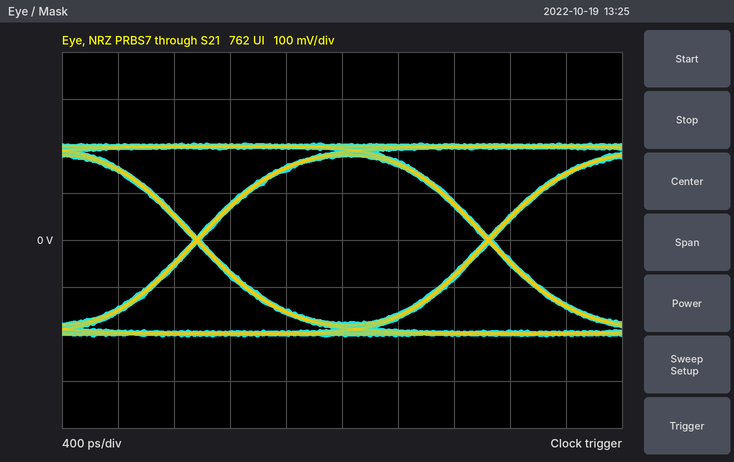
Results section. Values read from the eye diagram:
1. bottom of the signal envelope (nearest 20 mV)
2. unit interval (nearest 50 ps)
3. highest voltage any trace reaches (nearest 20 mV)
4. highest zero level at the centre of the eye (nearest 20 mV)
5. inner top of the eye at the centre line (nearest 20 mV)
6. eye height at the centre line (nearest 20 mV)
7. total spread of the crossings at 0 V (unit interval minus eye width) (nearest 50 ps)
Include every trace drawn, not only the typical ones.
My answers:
-200 mV
2.10 ns
200 mV
-180 mV
180 mV
360 mV
50 ps
